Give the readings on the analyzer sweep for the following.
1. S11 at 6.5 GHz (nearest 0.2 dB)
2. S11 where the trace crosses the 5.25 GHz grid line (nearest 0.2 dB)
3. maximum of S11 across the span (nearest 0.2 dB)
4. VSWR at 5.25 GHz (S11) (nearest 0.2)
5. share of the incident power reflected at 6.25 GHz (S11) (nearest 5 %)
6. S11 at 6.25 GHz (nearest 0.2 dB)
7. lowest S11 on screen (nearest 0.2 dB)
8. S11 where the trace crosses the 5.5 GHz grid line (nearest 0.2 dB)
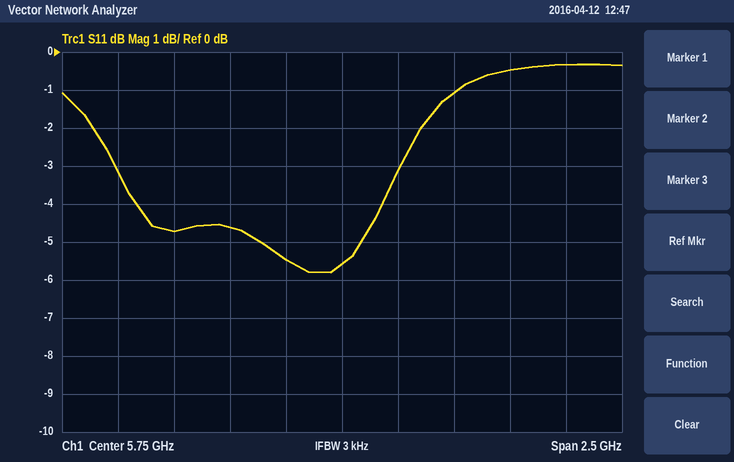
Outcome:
-0.4 dB
-4.6 dB
-0.4 dB
3.8
80 %
-1.0 dB
-5.8 dB
-5.4 dB
